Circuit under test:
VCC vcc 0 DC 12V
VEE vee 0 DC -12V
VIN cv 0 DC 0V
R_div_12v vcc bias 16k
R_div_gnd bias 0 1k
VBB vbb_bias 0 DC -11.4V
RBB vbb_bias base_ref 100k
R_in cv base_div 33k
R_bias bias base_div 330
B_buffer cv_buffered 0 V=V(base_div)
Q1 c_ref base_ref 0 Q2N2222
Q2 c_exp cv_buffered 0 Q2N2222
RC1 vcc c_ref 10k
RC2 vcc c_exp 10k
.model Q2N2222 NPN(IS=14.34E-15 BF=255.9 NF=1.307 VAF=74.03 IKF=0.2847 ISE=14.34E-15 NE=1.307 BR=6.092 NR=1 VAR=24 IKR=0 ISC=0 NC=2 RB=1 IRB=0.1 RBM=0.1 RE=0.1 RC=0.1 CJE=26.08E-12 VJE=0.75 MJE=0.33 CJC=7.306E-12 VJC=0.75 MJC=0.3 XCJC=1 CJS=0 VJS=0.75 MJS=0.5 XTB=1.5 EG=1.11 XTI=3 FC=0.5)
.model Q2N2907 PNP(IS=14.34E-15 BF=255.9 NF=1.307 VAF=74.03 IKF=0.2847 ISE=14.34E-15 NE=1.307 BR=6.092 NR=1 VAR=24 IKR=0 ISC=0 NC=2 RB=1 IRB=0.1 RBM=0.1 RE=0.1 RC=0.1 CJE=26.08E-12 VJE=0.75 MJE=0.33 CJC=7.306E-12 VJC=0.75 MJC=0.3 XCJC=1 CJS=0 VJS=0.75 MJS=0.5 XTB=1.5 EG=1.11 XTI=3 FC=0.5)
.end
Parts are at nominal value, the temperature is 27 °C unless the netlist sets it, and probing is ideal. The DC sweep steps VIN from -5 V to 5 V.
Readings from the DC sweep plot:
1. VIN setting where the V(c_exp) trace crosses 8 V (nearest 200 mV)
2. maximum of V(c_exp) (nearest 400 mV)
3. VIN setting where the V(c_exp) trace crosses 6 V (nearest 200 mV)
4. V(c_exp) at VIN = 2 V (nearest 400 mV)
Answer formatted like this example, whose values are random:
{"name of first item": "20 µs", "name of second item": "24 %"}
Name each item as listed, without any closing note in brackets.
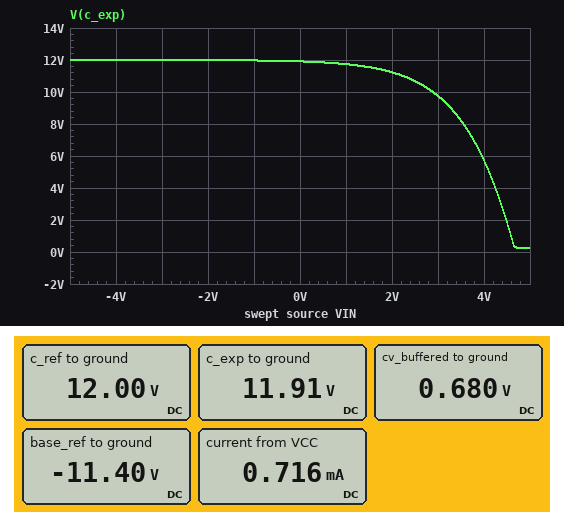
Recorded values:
{"VIN setting where the V(c_exp) trace crosses 8 V": "3.6 V", "maximum of V(c_exp)": "12.0 V", "VIN setting where the V(c_exp) trace crosses 6 V": "4.0 V", "V(c_exp) at VIN = 2 V": "11.2 V"}
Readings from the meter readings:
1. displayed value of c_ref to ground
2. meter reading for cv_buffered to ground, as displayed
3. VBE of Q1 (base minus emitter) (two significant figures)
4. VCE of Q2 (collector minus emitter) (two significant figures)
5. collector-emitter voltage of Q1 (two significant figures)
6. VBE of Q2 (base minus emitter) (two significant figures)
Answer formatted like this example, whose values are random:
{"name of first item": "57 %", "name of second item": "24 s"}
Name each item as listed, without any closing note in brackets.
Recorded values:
{"displayed value of c_ref to ground": "12.00 V", "meter reading for cv_buffered to ground, as displayed": "0.680 V", "VBE of Q1 (base minus emitter)": "-11 V", "VCE of Q2 (collector minus emitter)": "12 V", "collector-emitter voltage of Q1": "12 V", "VBE of Q2 (base minus emitter)": "680 mV"}
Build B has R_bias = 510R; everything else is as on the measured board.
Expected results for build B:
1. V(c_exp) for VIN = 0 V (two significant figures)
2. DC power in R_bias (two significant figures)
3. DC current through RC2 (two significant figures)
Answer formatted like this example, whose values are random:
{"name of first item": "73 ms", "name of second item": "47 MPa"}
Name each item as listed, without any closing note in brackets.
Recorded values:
{"V(c_exp) for VIN = 0 V": "12 V", "DC power in R_bias": "210 nW", "DC current through RC2": "7.8 µA"}
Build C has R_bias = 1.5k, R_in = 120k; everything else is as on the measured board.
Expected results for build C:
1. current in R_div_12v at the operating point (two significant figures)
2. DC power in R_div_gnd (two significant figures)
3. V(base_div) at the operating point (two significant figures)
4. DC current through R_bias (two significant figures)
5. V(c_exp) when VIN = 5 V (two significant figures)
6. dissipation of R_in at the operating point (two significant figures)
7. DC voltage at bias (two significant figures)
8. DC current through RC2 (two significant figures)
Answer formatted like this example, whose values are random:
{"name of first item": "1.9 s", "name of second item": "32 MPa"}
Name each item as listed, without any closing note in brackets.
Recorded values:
{"current in R_div_12v at the operating point": "710 µA", "DC power in R_div_gnd": "490 µW", "V(base_div) at the operating point": "690 mV", "DC current through R_bias": "5.8 µA", "V(c_exp) when VIN = 5 V": "9.7 V", "dissipation of R_in at the operating point": "4.0 µW", "DC voltage at bias": "700 mV", "DC current through RC2": "12 µA"}
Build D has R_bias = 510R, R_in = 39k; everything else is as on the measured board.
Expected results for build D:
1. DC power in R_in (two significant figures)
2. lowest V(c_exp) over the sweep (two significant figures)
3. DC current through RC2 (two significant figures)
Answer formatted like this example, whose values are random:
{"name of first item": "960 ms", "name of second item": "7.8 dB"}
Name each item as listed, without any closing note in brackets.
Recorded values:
{"DC power in R_in": "12 µW", "lowest V(c_exp) over the sweep": "250 mV", "DC current through RC2": "8.9 µA"}
